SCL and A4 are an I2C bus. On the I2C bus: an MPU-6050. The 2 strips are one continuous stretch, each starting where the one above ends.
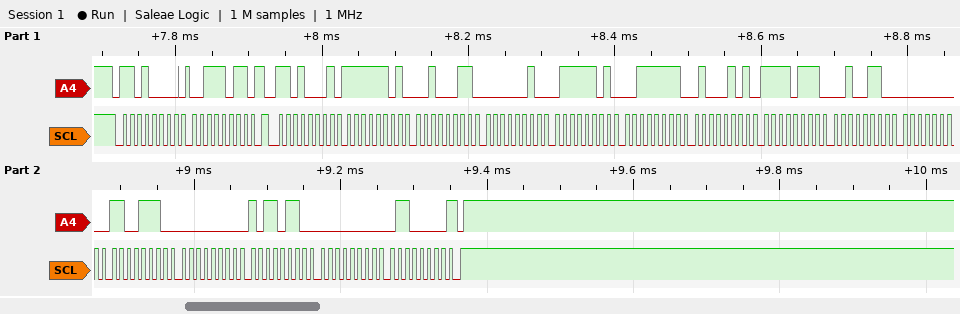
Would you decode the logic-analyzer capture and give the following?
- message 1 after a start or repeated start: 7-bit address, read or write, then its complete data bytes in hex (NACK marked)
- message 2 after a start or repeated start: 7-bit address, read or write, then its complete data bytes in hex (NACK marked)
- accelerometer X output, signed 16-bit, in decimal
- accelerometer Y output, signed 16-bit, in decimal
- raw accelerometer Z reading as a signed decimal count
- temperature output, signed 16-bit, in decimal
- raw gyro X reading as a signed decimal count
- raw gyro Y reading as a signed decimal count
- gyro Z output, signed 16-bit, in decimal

0x68 write: 3B
0x68 read: FD 23 02 7D 3F 45 F7 26 00 CE 00 B6 00 60 NACK
-733
637
16197
-2266
206
182
96
